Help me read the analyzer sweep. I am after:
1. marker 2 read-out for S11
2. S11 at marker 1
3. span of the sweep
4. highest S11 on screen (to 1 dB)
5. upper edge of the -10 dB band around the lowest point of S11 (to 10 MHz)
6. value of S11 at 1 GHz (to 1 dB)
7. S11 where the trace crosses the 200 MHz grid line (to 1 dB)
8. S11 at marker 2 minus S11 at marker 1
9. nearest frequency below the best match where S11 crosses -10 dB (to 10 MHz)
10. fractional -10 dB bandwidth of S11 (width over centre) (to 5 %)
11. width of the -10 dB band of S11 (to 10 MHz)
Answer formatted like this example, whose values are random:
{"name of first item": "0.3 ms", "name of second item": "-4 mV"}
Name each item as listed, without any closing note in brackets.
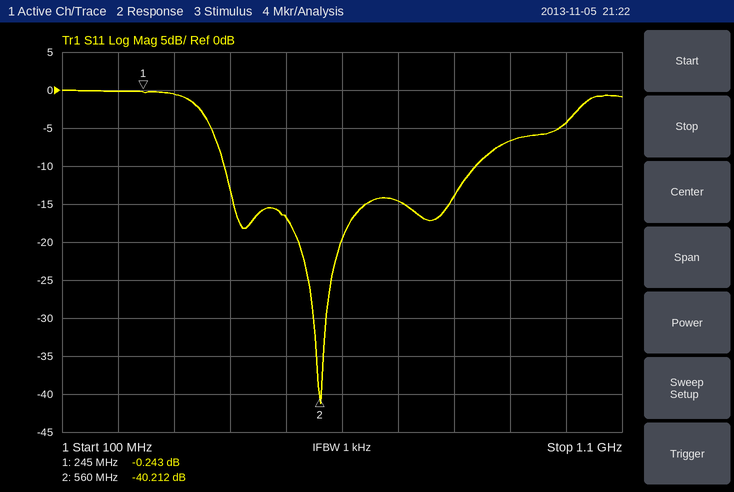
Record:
{"marker 2 read-out for S11": "-40.212 dB", "S11 at marker 1": "-0.243 dB", "span of the sweep": "1 GHz", "highest S11 on screen": "0 dB", "upper edge of the -10 dB band around the lowest point of S11": "840 MHz", "value of S11 at 1 GHz": "-4 dB", "S11 where the trace crosses the 200 MHz grid line": "0 dB", "S11 at marker 2 minus S11 at marker 1": "-39.969 dB", "nearest frequency below the best match where S11 crosses -10 dB": "390 MHz", "fractional -10 dB bandwidth of S11 (width over centre)": "75 %", "width of the -10 dB band of S11": "450 MHz"}
